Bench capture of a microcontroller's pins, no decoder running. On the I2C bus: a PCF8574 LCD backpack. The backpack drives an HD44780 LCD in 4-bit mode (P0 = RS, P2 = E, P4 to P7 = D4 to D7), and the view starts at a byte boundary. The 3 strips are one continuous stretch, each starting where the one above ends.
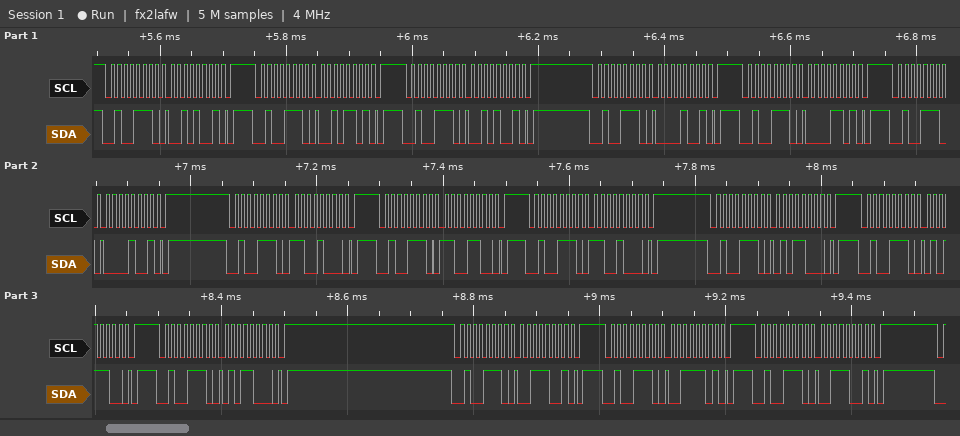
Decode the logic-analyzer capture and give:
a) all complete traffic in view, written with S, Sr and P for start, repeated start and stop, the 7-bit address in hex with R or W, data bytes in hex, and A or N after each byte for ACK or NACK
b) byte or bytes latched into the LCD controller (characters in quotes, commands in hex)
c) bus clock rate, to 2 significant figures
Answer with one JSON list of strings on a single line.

["S 27W A 29 A P S 27W A 2D A P S 27W A 29 A P S 27W A 09 A P S 27W A 0D A P S 27W A 09 A P S 27W A C8 A P S 27W A CC A P S 27W A C8 A P S 27W A 58 A P S 27W A 5C A P S 27W A 58 A P S 27W A 39 A P S 27W A 3D A P S 27W A 39 A P", "' ' 0xC5", "100 kHz"]
